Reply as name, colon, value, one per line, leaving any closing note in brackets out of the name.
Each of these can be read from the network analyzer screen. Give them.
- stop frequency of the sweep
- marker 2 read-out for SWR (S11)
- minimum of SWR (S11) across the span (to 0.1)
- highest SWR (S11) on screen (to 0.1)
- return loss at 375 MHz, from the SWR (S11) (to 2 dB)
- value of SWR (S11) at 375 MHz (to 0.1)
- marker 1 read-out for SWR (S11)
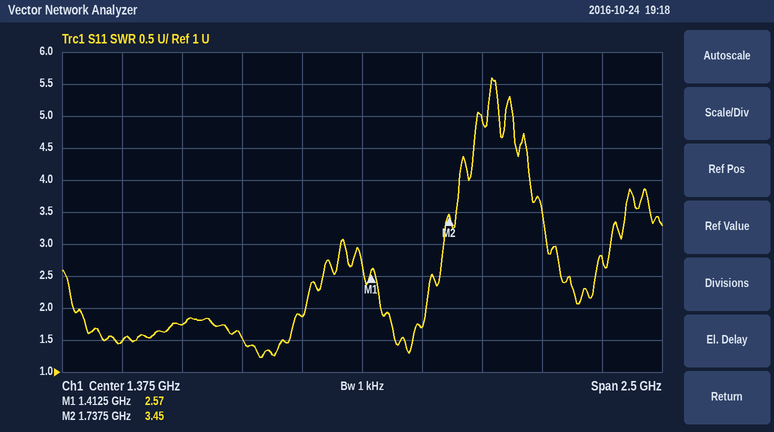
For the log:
stop frequency of the sweep: 2.625 GHz
marker 2 read-out for SWR: 3.45
minimum of SWR (S11) across the span: 1.2
highest SWR (S11) on screen: 5.6
return loss at 375 MHz, from the SWR (S11): 14 dB
value of SWR (S11) at 375 MHz: 1.5
marker 1 read-out for SWR: 2.57
